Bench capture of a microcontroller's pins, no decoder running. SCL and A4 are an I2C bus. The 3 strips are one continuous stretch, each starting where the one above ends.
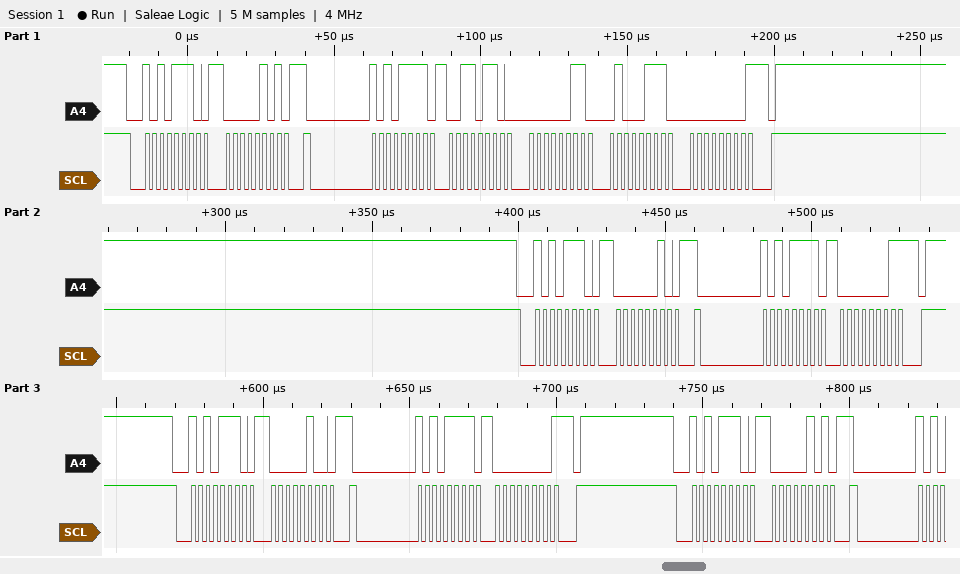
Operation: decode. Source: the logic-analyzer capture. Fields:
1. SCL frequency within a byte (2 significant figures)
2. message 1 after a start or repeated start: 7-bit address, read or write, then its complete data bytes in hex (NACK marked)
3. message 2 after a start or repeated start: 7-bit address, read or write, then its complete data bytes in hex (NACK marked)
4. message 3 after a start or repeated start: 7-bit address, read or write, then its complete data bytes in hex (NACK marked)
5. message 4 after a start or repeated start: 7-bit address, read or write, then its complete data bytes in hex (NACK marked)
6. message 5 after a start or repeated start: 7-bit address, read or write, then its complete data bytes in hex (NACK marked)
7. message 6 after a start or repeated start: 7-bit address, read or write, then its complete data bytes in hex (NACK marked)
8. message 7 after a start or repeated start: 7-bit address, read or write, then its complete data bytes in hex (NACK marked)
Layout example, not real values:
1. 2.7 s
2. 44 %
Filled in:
1. 400 kHz
2. 0x57 write: 05
3. 0x57 read: 36 03 47 00 NACK
4. 0x57 write: 02
5. 0x57 read: 01 NACK
6. 0x57 write: 04
7. 0x57 read: 00 NACK
8. 0x57 write: 05
